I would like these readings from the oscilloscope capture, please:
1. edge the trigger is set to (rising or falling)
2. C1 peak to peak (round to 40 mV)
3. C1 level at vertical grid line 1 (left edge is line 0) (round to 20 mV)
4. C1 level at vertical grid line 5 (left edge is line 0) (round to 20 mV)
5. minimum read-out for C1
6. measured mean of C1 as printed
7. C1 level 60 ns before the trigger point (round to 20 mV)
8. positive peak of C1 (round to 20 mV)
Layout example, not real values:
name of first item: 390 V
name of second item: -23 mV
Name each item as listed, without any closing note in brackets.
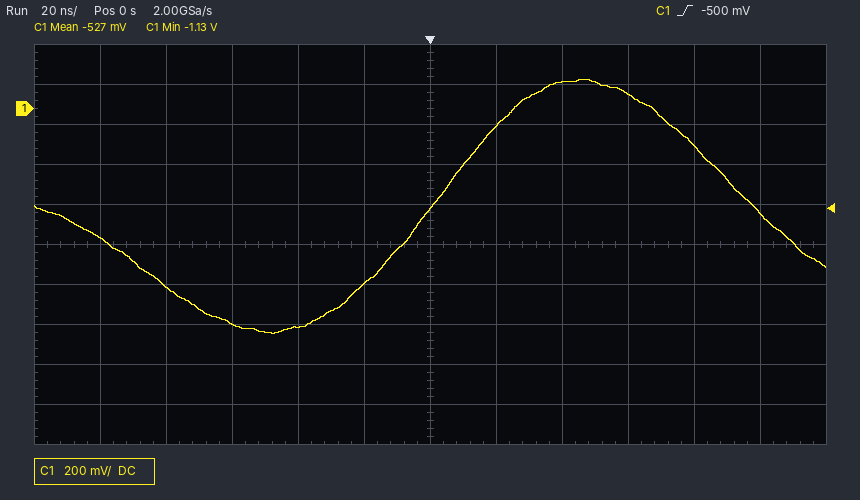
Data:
edge the trigger is set to: rising
C1 peak to peak: 1.28 V
C1 level at vertical grid line 1 (left edge is line 0): -640 mV
C1 level at vertical grid line 5 (left edge is line 0): -880 mV
minimum read-out for C1: -1.13 V
measured mean of C1 as printed: -527 mV
C1 level 60 ns before the trigger point: -1.08 V
positive peak of C1: 140 mV
